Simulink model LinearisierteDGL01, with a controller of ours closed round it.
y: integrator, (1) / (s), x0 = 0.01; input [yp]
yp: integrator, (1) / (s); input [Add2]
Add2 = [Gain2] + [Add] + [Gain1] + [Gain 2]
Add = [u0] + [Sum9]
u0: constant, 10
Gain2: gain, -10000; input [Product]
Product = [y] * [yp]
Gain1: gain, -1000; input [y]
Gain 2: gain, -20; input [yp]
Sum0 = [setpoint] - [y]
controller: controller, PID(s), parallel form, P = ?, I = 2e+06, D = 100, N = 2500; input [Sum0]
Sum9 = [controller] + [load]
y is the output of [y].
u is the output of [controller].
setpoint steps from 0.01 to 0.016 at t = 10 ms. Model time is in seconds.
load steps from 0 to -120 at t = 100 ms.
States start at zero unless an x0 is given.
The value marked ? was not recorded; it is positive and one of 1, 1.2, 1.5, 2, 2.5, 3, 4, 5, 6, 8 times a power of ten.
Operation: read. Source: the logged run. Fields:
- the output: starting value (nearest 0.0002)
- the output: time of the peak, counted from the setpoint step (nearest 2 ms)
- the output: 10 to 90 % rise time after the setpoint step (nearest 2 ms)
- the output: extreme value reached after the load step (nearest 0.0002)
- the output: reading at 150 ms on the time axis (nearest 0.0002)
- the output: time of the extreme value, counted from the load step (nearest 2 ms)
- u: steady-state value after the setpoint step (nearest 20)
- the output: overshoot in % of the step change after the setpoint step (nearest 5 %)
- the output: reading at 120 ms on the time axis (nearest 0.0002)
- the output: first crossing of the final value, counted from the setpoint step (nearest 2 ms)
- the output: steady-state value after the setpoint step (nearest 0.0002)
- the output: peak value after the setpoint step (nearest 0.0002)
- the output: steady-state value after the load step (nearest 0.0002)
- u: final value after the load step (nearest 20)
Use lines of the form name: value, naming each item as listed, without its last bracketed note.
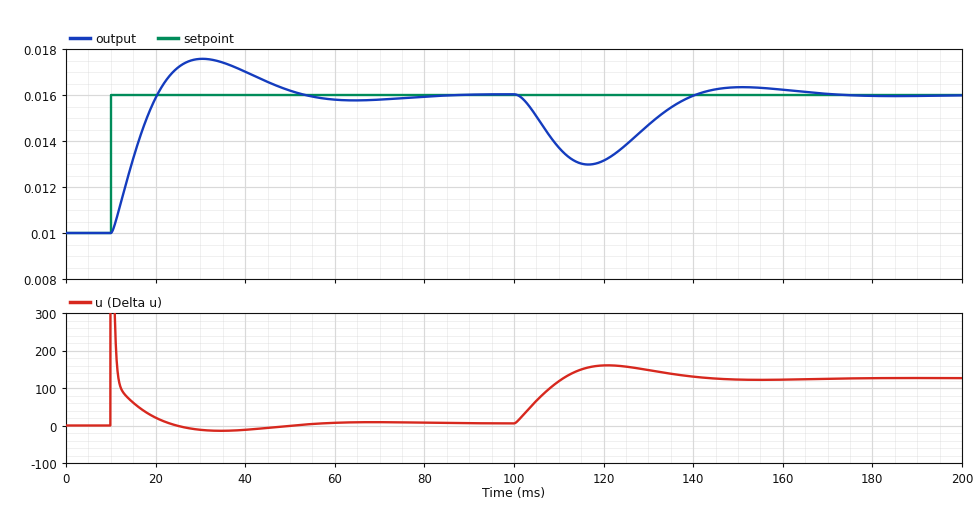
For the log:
the output: starting value: 0.0100
the output: time of the peak, counted from the setpoint step: 20 ms
the output: 10 to 90 % rise time after the setpoint step: 8 ms
the output: extreme value reached after the load step: 0.0130
the output: reading at 150 ms on the time axis: 0.0164
the output: time of the extreme value, counted from the load step: 16 ms
u: steady-state value after the setpoint step: 0
the output: overshoot in % of the step change after the setpoint step: 25 %
the output: reading at 120 ms on the time axis: 0.0132
the output: first crossing of the final value, counted from the setpoint step: 10 ms
the output: steady-state value after the setpoint step: 0.0160
the output: peak value after the setpoint step: 0.0176
the output: steady-state value after the load step: 0.0160
u: final value after the load step: 120
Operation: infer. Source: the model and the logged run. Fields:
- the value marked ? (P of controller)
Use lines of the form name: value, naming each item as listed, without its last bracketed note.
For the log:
the value marked ?: 30000
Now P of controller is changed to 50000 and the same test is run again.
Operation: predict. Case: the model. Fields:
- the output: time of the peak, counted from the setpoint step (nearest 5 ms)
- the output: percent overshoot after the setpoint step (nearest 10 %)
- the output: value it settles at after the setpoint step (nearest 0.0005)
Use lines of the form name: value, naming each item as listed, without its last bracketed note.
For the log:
the output: time of the peak, counted from the setpoint step: 15 ms
the output: percent overshoot after the setpoint step: 20 %
the output: value it settles at after the setpoint step: 0.0160
